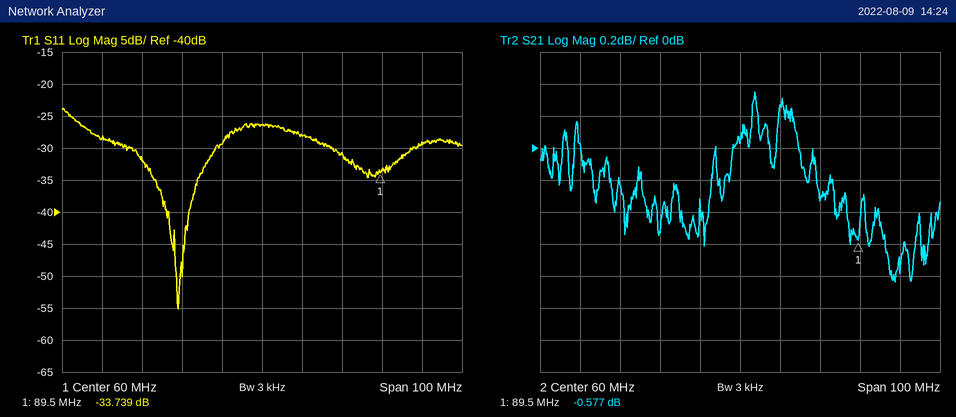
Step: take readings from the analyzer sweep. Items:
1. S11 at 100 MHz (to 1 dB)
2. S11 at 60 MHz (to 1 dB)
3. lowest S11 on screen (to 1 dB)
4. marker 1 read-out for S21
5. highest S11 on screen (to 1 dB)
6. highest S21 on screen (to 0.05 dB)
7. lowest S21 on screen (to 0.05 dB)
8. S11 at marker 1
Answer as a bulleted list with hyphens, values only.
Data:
- -29 dB
- -26 dB
- -55 dB
- -0.577 dB
- -24 dB
- 0.35 dB
- -0.85 dB
- -33.739 dB
